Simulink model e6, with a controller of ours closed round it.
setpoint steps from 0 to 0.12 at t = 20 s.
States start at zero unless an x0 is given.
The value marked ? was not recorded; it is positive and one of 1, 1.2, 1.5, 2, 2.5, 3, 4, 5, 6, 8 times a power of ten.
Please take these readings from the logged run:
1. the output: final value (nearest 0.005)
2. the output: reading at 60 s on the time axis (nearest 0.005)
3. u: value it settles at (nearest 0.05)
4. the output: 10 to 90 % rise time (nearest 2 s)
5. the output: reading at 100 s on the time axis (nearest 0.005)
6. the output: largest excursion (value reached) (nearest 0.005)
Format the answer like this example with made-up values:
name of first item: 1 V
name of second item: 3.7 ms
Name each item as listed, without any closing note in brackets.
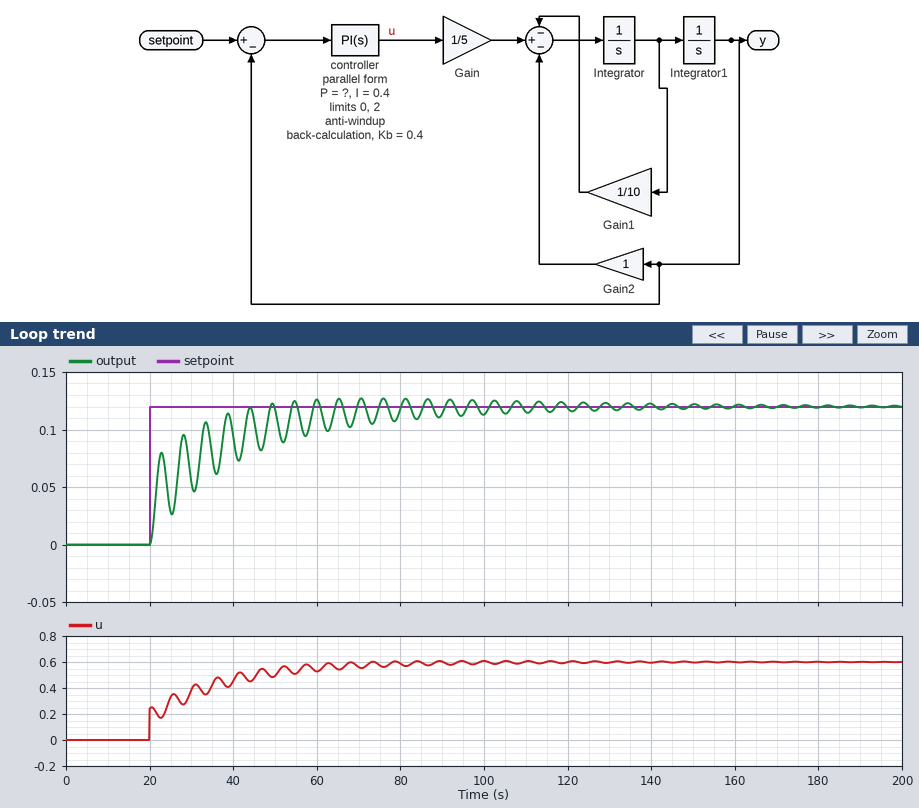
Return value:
the output: final value: 0.120
the output: reading at 60 s on the time axis: 0.125
u: value it settles at: 0.60
the output: 10 to 90 % rise time: 18 s
the output: reading at 100 s on the time axis: 0.115
the output: largest excursion (value reached): 0.125
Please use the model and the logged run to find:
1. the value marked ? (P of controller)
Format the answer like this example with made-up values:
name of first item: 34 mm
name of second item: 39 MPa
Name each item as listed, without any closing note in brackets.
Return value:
the value marked ?: 2
